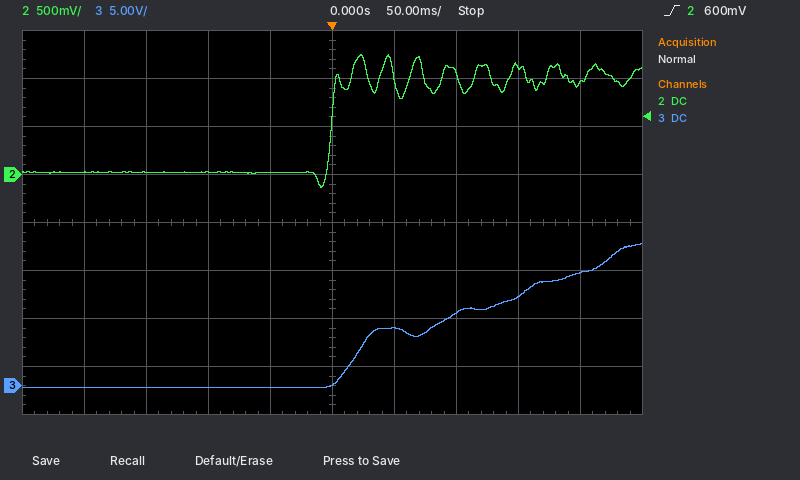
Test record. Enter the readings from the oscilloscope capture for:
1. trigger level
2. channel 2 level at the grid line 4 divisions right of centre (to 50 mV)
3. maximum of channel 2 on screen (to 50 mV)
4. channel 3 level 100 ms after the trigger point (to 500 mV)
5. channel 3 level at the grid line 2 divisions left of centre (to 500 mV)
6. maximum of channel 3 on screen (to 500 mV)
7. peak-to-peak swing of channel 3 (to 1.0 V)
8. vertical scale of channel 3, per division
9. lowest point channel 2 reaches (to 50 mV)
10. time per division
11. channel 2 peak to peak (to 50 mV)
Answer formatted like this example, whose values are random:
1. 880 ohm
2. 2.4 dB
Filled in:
1. 600 mV
2. 950 mV
3. 1.25 V
4. 7.5 V
5. 0.0 V
6. 15.0 V
7. 15.0 V
8. 5 V
9. -150 mV
10. 50 ms
11. 1.40 V
